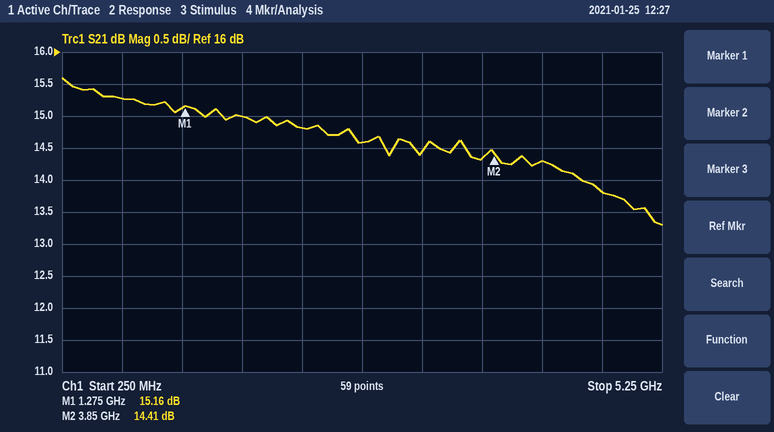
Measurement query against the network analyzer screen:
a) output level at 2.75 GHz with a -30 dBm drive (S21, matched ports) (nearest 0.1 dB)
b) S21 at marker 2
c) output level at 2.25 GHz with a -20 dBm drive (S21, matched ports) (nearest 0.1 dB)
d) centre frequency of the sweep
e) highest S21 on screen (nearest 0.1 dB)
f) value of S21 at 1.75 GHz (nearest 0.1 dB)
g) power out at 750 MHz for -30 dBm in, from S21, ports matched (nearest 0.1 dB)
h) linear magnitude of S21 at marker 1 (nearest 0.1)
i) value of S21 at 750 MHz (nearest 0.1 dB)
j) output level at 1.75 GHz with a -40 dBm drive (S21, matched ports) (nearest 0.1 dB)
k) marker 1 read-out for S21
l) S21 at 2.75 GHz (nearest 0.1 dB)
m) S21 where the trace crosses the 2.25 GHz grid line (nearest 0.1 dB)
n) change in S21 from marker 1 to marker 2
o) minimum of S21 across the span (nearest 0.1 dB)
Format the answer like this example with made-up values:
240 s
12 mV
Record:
-15.4 dBm
14.41 dB
-5.2 dBm
2.75 GHz
15.6 dB
15.0 dB
-14.7 dBm
5.7
15.3 dB
-25.0 dBm
15.16 dB
14.6 dB
14.8 dB
-0.75 dB
13.3 dB
